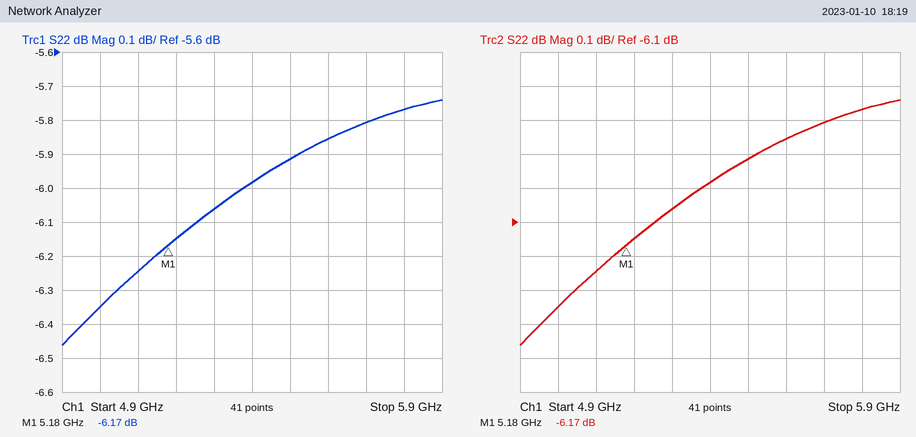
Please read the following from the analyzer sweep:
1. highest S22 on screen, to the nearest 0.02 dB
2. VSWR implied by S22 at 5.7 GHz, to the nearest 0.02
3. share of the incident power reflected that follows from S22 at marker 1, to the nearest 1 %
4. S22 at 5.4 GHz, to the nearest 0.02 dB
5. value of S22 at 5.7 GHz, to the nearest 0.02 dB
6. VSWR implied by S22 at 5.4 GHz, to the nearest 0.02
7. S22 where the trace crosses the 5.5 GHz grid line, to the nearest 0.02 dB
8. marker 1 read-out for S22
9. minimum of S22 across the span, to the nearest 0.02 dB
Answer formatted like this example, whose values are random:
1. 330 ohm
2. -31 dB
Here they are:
1. -5.74 dB
2. 3.10
3. 24 %
4. -5.98 dB
5. -5.80 dB
6. 3.02
7. -5.92 dB
8. -6.17 dB
9. -6.46 dB
